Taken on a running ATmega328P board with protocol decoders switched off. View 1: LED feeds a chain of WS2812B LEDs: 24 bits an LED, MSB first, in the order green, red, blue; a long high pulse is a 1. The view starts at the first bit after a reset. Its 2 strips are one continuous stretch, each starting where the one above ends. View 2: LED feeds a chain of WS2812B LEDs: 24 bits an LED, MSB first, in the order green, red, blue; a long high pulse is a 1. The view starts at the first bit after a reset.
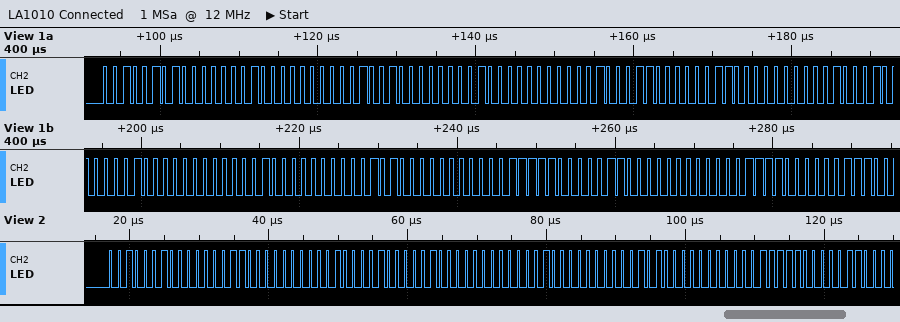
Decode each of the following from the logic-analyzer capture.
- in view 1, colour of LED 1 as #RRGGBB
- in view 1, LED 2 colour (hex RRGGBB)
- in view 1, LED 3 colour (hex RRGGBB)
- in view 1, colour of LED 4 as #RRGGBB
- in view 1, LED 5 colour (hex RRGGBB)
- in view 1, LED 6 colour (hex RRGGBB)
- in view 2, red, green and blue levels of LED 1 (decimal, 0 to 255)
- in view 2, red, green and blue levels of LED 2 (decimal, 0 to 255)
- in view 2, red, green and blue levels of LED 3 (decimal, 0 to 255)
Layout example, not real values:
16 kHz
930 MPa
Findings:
#012500
#022400
#032300
#042200
#052000
#061F00
3, 34, 0
4, 33, 0
5, 32, 0
